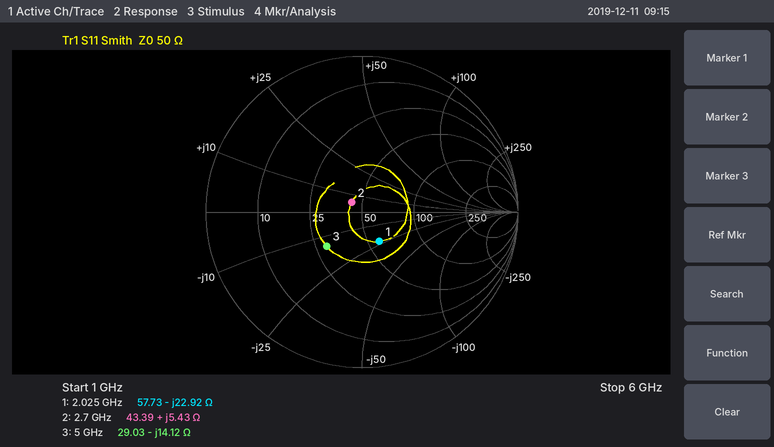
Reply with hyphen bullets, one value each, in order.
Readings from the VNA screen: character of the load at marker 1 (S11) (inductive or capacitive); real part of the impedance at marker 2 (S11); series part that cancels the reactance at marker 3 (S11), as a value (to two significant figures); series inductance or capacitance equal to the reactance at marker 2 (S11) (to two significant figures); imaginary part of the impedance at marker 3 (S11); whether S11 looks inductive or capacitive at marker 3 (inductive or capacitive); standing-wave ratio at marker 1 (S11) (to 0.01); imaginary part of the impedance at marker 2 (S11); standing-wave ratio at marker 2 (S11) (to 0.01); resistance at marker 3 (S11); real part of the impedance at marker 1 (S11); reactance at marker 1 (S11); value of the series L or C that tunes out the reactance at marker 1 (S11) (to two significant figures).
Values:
- capacitive
- 43.39 Ω
- 450 pH
- 320 pH
- -14.12 Ω
- capacitive
- 1.56
- +5.43 Ω
- 1.20
- 29.03 Ω
- 57.73 Ω
- -22.92 Ω
- 1.8 nH
